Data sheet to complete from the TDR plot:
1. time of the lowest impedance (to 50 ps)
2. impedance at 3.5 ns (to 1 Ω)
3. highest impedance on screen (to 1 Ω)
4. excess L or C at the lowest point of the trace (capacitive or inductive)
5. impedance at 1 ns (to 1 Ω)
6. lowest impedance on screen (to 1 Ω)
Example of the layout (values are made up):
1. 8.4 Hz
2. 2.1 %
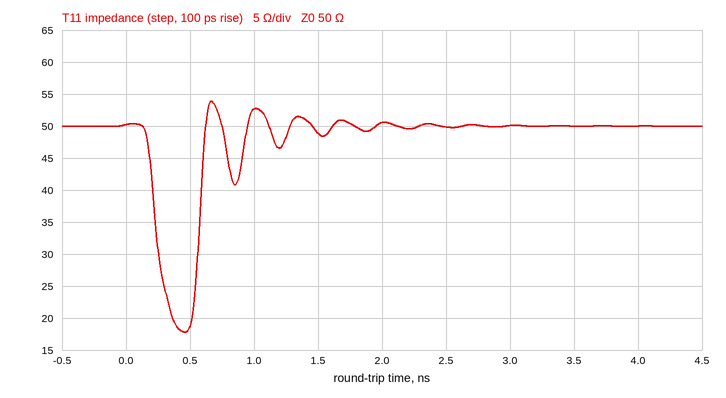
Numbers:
1. 450 ps
2. 50 Ω
3. 54 Ω
4. capacitive
5. 53 Ω
6. 18 Ω
